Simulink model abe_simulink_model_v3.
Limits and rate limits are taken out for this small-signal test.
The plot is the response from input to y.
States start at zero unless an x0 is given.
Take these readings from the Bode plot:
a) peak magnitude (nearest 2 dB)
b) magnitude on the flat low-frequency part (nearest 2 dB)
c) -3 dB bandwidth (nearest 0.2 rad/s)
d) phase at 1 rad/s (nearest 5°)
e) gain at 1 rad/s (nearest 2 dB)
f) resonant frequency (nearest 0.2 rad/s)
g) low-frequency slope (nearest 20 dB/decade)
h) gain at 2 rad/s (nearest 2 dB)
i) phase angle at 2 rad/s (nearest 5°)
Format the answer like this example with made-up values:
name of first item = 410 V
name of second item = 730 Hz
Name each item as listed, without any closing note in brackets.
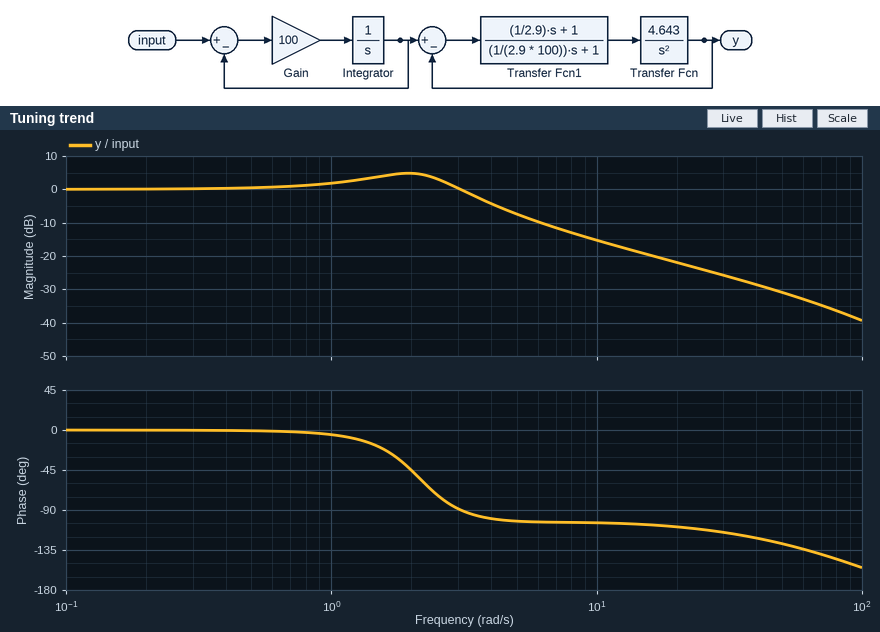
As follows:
peak magnitude = 4 dB
magnitude on the flat low-frequency part = 0 dB
-3 dB bandwidth = 3.6 rad/s
phase at 1 rad/s = -5°
gain at 1 rad/s = 2 dB
resonant frequency = 2.0 rad/s
low-frequency slope = 0 dB/decade
gain at 2 rad/s = 4 dB
phase angle at 2 rad/s = -45°
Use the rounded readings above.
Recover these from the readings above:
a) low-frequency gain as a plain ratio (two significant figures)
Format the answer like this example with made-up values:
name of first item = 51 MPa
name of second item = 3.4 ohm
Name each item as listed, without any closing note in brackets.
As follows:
low-frequency gain as a plain ratio = 1.0
